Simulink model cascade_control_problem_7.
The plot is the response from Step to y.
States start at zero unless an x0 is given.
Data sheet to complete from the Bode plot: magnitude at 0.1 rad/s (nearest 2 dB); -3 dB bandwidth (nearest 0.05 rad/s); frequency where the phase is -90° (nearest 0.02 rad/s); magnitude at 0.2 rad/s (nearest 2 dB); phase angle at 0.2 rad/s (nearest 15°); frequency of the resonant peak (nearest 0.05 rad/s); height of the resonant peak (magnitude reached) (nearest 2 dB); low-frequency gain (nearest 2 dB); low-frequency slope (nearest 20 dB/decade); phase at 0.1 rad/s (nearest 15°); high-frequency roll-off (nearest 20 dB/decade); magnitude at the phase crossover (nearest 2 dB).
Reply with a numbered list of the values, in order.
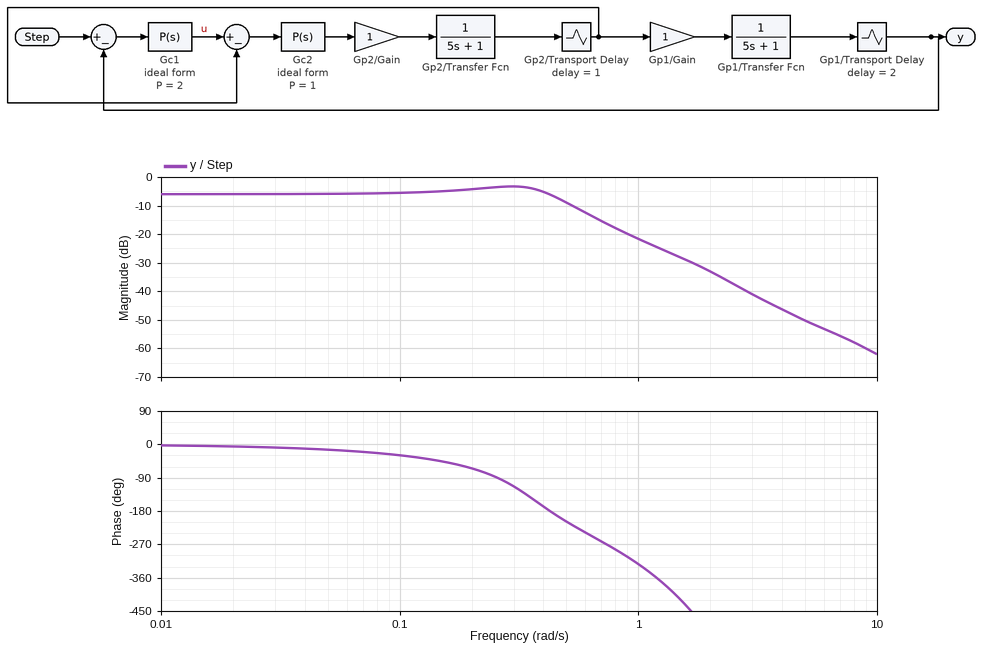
1. -6 dB
2. 0.50 rad/s
3. 0.26 rad/s
4. -4 dB
5. -60°
6. 0.30 rad/s
7. -4 dB
8. -6 dB
9. 0 dB/decade
10. -30°
11. -40 dB/decade
12. -6 dB
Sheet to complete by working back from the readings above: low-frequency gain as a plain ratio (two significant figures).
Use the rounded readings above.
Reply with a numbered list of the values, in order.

1. 0.50
